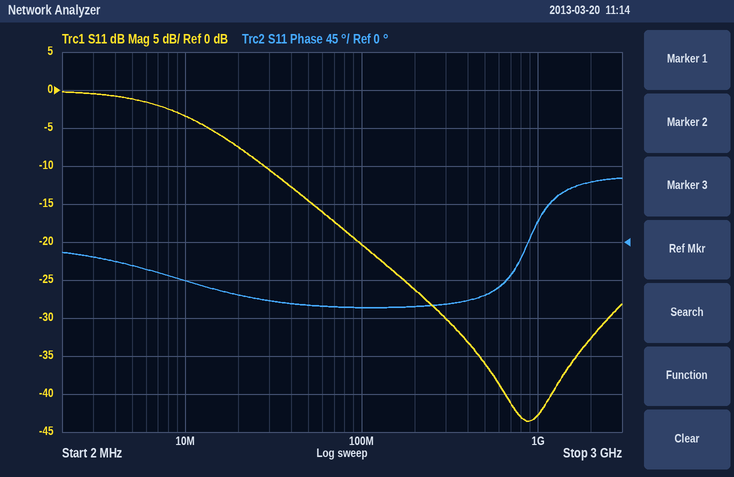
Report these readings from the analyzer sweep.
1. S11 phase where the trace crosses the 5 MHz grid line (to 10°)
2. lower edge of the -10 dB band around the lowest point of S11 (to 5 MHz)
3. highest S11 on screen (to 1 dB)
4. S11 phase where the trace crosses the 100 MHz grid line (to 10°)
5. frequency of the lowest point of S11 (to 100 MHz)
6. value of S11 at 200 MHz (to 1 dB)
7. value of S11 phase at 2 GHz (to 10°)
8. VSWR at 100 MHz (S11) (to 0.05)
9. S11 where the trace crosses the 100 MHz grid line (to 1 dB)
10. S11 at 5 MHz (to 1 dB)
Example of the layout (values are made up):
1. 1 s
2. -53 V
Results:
1. -30°
2. 30 MHz
3. 0 dB
4. -80°
5. 900 MHz
6. -26 dB
7. 70°
8. 1.20
9. -20 dB
10. -1 dB
